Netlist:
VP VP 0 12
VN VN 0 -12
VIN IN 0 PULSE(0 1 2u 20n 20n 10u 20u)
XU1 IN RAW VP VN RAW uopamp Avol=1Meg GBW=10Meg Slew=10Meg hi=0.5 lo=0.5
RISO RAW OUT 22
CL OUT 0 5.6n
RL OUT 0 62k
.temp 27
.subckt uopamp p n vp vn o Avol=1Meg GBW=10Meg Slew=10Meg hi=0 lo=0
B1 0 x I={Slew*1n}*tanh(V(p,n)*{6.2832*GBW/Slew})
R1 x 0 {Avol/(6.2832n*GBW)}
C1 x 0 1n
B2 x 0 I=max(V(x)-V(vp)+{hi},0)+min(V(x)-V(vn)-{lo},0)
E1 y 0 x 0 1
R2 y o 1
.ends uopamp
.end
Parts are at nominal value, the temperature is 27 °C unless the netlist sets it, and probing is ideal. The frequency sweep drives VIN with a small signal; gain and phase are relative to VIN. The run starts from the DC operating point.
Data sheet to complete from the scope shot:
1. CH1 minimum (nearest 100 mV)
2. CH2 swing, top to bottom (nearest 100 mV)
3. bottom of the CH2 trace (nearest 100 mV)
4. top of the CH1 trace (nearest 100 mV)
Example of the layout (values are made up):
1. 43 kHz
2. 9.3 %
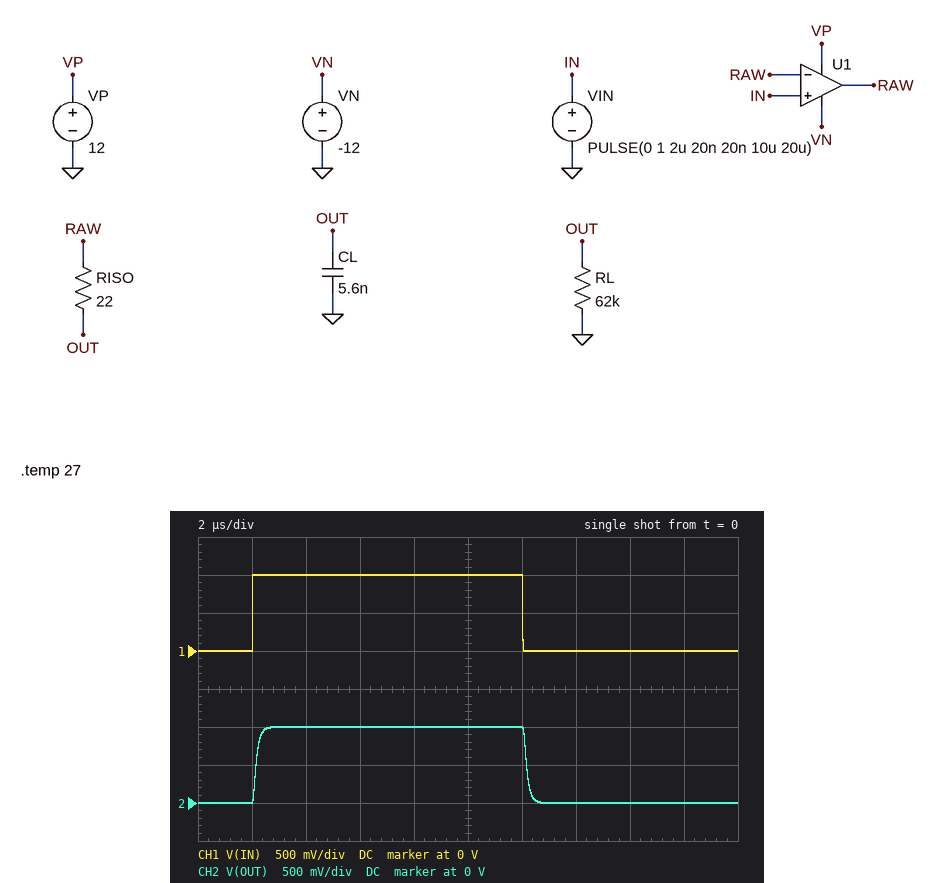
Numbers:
1. 0 V
2. 1.0 V
3. 0 V
4. 1.0 V
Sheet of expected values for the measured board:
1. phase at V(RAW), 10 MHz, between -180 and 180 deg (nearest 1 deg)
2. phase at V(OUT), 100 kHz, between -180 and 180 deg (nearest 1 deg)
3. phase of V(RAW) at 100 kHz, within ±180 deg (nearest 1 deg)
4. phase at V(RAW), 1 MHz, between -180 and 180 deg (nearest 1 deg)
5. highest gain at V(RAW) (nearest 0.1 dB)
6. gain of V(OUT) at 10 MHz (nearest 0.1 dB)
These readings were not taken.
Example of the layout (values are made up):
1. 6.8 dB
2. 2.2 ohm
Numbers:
1. -46 deg
2. -5 deg
3. -1 deg
4. -6 deg
5. 0 dB
6. -21.0 dB
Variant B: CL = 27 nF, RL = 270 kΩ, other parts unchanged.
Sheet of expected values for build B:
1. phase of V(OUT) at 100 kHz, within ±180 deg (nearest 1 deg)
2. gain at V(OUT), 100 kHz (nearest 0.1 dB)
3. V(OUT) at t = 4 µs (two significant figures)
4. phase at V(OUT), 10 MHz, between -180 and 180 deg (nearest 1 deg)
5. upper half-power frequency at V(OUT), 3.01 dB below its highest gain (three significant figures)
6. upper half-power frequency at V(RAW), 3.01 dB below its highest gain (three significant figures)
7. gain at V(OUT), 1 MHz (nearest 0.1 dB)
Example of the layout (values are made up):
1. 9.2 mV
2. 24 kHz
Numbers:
1. -21 deg
2. -0.6 dB
3. 960 mV
4. -135 deg
5. 268 kHz
6. 9.57 MHz
7. -11.8 dB
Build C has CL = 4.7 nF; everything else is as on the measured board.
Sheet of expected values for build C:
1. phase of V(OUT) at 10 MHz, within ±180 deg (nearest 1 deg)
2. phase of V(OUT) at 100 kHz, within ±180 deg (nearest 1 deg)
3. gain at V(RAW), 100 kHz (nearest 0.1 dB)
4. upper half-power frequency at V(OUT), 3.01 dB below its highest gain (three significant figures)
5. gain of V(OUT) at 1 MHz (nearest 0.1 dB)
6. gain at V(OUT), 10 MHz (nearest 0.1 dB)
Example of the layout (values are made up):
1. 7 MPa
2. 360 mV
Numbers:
1. -128 deg
2. -4 deg
3. 0 dB
4. 1.51 MHz
5. -1.6 dB
6. -19.5 dB
